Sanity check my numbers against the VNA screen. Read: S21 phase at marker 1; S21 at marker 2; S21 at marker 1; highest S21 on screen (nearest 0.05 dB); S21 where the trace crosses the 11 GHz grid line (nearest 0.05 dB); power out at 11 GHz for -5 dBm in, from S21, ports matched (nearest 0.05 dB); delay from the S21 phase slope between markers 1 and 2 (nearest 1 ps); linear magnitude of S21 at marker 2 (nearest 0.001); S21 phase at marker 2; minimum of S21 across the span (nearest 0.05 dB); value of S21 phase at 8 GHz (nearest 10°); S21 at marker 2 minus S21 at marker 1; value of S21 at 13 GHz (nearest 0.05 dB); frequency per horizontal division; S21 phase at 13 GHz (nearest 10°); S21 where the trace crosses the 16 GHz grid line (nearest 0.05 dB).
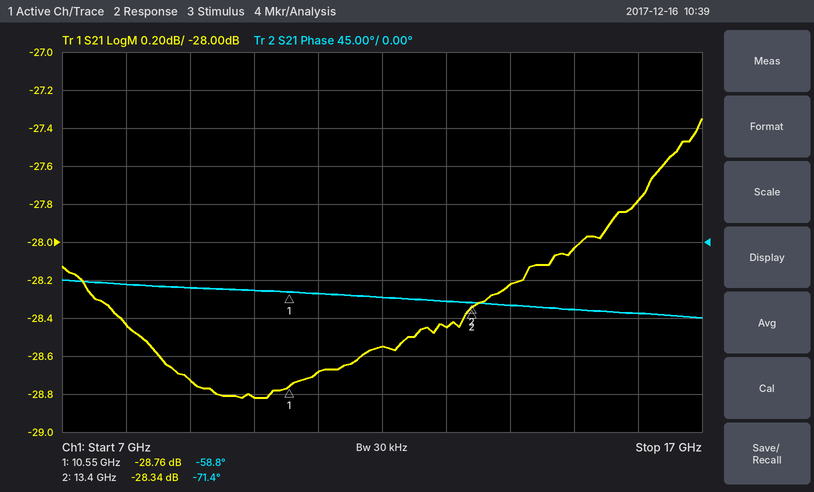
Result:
-58.8°
-28.34 dB
-28.76 dB
-27.35 dB
-28.70 dB
-33.70 dBm
12 ps
0.038
-71.4°
-28.80 dB
-50°
0.42 dB
-28.45 dB
1 GHz
-70°
-27.80 dB
